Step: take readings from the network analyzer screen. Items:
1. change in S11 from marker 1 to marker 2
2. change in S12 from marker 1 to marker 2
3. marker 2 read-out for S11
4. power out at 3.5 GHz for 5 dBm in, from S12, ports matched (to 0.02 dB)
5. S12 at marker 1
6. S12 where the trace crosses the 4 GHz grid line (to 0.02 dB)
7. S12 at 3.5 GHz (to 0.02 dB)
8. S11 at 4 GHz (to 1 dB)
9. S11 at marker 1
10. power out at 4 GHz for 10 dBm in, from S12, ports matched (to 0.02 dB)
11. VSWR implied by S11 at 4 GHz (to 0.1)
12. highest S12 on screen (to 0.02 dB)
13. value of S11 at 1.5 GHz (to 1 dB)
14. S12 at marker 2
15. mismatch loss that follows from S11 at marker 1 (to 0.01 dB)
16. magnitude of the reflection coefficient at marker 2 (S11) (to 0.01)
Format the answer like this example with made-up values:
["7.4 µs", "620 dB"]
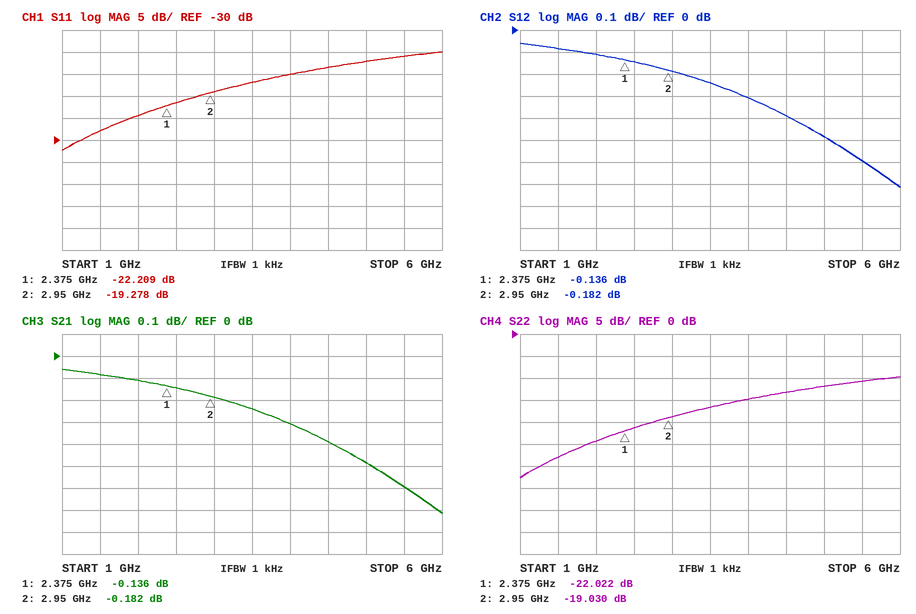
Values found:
["2.931 dB", "-0.046 dB", "-19.278 dB", "4.76 dBm", "-0.136 dB", "-0.30 dB", "-0.24 dB", "-15 dB", "-22.209 dB", "9.70 dBm", "1.4", "-0.06 dB", "-28 dB", "-0.182 dB", "0.03 dB", "0.11"]
